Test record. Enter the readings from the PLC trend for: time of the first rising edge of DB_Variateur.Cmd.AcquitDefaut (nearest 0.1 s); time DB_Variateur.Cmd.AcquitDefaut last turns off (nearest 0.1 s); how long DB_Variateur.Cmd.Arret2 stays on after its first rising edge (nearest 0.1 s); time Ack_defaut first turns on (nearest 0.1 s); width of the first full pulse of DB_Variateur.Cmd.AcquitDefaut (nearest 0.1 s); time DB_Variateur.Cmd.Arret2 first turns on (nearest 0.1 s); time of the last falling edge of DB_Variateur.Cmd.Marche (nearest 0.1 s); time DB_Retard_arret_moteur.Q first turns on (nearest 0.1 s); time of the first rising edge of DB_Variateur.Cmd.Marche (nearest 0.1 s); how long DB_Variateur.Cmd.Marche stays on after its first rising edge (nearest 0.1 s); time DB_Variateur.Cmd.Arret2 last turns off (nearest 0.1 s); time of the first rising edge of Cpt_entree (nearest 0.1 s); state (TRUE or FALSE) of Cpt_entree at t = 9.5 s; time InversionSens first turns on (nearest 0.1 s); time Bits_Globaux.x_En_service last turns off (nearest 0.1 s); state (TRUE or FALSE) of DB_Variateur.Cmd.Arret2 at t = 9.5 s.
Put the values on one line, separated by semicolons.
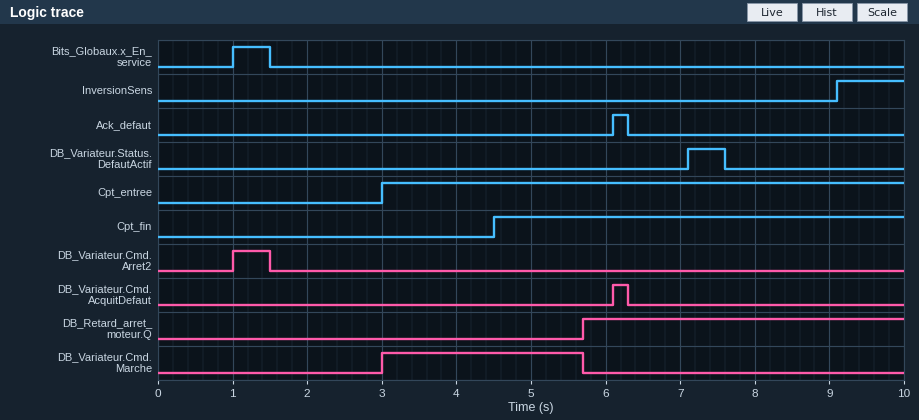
6.1 s; 6.3 s; 0.5 s; 6.1 s; 0.2 s; 1.0 s; 5.7 s; 5.7 s; 3.0 s; 2.7 s; 1.5 s; 3.0 s; TRUE; 9.1 s; 1.5 s; FALSE
